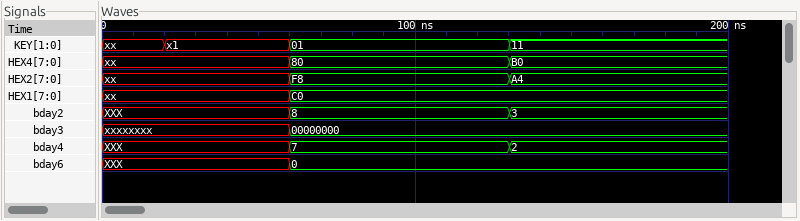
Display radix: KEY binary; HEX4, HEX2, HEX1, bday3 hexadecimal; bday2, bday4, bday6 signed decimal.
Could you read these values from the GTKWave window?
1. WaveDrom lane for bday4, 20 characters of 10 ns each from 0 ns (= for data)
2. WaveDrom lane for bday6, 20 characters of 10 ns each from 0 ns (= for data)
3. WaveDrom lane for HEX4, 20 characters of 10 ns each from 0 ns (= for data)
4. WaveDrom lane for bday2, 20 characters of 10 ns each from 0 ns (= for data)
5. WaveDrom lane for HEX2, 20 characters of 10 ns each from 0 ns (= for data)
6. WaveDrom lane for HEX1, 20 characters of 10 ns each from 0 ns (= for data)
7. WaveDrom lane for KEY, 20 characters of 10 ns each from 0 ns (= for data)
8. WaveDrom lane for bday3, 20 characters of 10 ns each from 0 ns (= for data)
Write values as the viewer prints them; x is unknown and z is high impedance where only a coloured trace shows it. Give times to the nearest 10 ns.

{name: 'bday4', wave: 'x.....=......=......', data: '7 2'}
{name: 'bday6', wave: 'x.....=.............', data: '0'}
{name: 'HEX4', wave: 'x.....=......=......', data: '80 B0'}
{name: 'bday2', wave: 'x.....=......=......', data: '8 3'}
{name: 'HEX2', wave: 'x.....=......=......', data: 'F8 A4'}
{name: 'HEX1', wave: 'x.....=.............', data: 'C0'}
{name: 'KEY', wave: 'x.=...=......=......', data: 'x1 01 11'}
{name: 'bday3', wave: 'x.....=.............', data: '00000000'}
